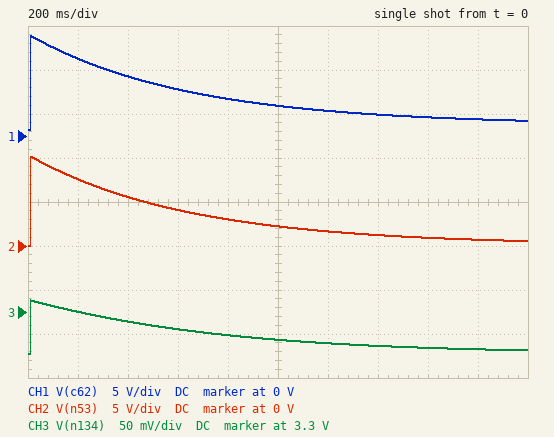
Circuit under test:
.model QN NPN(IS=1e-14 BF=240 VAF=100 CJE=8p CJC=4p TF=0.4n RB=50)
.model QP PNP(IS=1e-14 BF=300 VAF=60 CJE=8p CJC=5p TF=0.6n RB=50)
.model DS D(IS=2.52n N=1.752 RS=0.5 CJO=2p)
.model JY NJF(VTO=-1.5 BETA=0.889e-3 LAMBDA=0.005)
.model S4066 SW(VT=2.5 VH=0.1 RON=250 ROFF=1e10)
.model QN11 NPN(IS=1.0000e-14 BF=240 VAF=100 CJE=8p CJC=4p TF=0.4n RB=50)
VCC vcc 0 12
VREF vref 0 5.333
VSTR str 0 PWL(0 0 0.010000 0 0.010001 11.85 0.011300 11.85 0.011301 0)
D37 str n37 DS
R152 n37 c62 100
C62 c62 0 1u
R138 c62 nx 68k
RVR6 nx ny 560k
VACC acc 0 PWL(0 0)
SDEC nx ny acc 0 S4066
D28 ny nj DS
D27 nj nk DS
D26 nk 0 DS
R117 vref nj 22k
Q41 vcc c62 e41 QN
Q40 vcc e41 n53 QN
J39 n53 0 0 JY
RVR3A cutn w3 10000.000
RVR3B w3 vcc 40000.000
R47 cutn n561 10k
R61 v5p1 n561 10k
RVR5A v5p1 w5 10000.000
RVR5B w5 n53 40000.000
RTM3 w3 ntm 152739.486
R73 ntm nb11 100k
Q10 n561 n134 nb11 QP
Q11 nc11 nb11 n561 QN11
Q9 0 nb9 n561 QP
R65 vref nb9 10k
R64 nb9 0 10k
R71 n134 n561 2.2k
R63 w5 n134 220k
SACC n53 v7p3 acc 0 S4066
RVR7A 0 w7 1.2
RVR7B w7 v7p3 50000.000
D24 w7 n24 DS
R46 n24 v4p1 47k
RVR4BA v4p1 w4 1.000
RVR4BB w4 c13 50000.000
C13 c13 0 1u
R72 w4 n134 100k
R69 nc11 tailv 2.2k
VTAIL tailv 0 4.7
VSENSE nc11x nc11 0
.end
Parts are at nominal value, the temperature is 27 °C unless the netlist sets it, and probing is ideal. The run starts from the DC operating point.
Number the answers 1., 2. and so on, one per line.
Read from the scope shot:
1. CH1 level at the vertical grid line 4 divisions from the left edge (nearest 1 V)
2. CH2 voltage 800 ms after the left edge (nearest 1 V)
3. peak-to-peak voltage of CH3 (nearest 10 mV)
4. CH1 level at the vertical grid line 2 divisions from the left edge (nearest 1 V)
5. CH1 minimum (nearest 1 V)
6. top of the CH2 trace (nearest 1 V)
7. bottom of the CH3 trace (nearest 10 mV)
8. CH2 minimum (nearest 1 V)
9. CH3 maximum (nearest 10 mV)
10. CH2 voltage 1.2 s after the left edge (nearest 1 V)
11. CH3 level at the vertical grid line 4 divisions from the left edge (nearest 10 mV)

1. 4 V
2. 3 V
3. 60 mV
4. 7 V
5. 1 V
6. 10 V
7. 3.25 V
8. 0 V
9. 3.31 V
10. 2 V
11. 3.27 V
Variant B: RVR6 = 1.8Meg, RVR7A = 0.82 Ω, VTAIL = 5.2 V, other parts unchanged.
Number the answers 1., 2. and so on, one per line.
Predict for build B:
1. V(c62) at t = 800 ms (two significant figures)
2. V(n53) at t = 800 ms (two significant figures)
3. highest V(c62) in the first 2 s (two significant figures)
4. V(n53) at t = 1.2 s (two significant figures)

1. 7.9 V
2. 6.7 V
3. 11 V
4. 5.4 V
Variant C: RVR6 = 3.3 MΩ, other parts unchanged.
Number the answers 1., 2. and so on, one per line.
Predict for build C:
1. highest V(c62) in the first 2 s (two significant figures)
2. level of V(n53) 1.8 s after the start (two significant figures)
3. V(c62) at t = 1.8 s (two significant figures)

1. 11 V
2. 6.0 V
3. 7.2 V
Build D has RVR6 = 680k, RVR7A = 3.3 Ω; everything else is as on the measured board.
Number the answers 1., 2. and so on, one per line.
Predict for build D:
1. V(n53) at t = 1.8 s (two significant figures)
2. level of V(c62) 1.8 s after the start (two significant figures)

1. 1.0 V
2. 2.2 V
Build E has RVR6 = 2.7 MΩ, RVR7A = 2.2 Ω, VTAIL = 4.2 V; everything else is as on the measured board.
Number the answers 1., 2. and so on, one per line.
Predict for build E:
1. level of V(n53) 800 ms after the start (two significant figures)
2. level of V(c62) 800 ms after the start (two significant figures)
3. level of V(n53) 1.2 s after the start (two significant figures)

1. 7.7 V
2. 8.9 V
3. 6.6 V
